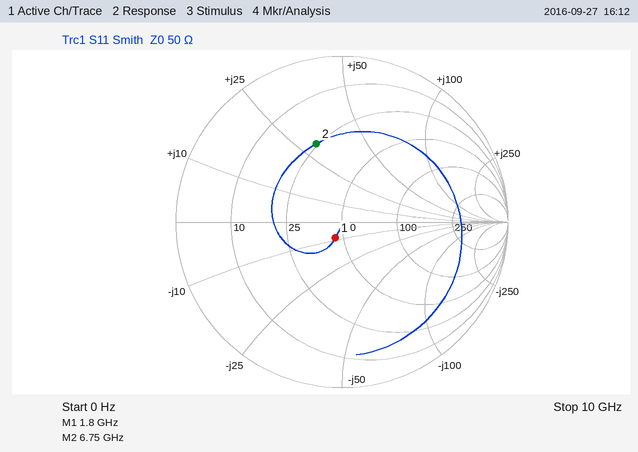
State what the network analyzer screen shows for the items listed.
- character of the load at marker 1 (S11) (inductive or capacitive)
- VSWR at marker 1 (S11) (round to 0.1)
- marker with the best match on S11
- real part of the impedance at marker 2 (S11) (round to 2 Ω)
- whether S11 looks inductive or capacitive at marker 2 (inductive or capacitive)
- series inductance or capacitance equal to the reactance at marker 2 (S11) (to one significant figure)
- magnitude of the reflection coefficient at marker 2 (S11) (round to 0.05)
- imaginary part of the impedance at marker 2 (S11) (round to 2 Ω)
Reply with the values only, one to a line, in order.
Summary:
capacitive
1.2
marker 1
24 Ω
inductive
700 pH
0.50
+30 Ω
